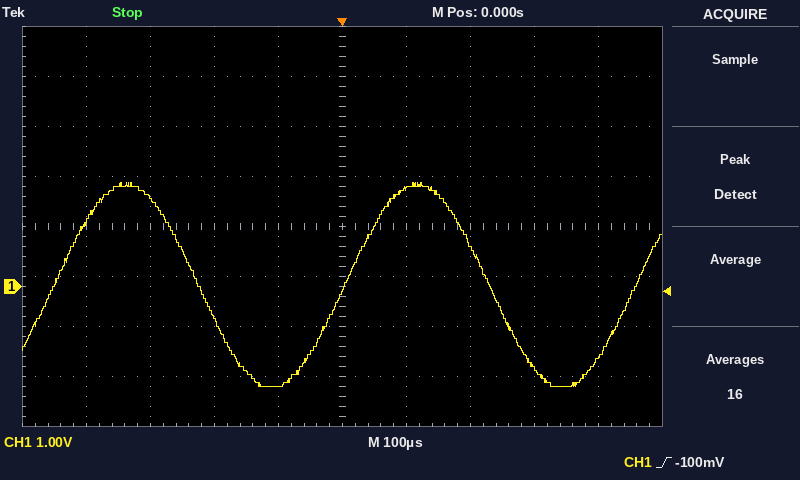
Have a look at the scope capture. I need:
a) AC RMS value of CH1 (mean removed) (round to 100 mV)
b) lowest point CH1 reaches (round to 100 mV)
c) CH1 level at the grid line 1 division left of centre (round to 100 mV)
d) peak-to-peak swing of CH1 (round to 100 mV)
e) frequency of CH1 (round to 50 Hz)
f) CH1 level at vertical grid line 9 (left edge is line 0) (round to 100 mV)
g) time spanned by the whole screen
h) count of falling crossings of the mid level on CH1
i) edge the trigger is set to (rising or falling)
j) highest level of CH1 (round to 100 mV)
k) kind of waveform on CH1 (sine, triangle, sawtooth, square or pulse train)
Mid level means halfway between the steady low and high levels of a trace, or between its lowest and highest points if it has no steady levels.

1.4 V
-2.0 V
-2.0 V
4.1 V
2.20 kHz
-1.4 V
1 ms
2
rising
2.1 V
sine
